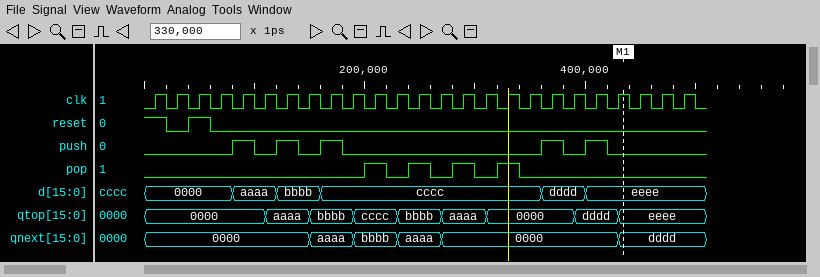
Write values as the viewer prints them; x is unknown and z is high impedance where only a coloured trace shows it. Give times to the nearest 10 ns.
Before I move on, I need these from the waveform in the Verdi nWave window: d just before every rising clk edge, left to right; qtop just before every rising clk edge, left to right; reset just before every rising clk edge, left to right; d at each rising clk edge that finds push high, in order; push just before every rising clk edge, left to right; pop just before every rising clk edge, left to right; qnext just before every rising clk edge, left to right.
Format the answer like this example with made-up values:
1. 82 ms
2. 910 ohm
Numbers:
1. 0000, 0000, 0000, 0000, aaaa, aaaa, bbbb, bbbb, cccc, cccc, cccc, cccc, cccc, cccc, cccc, cccc, cccc, cccc, dddd, dddd, eeee, eeee, eeee, eeee, eeee
2. 0000, 0000, 0000, 0000, 0000, 0000, aaaa, aaaa, bbbb, bbbb, cccc, cccc, bbbb, bbbb, aaaa, aaaa, 0000, 0000, 0000, 0000, dddd, dddd, eeee, eeee, eeee
3. 1 0 1 0 0 0 0 0 0 0 0 0 0 0 0 0 0 0 0 0 0 0 0 0 0
4. aaaa, bbbb, cccc, dddd, eeee
5. 0 0 0 0 1 0 1 0 1 0 0 0 0 0 0 0 0 0 1 0 1 0 0 0 0
6. 0 0 0 0 0 0 0 0 0 0 1 0 1 0 1 0 1 0 0 0 0 0 0 0 0
7. 0000, 0000, 0000, 0000, 0000, 0000, 0000, 0000, aaaa, aaaa, bbbb, bbbb, aaaa, aaaa, 0000, 0000, 0000, 0000, 0000, 0000, 0000, 0000, dddd, dddd, dddd
